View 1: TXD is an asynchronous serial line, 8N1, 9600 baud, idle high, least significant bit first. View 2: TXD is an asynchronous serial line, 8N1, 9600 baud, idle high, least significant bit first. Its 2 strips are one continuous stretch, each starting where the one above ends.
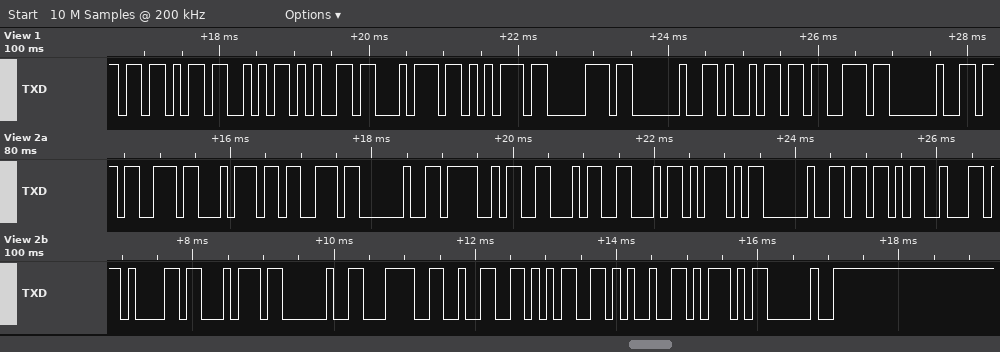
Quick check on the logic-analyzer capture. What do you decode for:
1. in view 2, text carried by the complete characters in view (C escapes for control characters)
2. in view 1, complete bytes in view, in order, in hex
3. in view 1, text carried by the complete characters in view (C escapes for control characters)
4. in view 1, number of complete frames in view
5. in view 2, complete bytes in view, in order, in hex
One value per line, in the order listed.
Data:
"sts OFF] [bat <25%] "
5B 53 65 74 75 70 20 69 73 20
"[Setup is "
10
73 74 73 20 4F 46 46 5D 20 5B 62 61 74 20 3C 32 35 25 5D 20
